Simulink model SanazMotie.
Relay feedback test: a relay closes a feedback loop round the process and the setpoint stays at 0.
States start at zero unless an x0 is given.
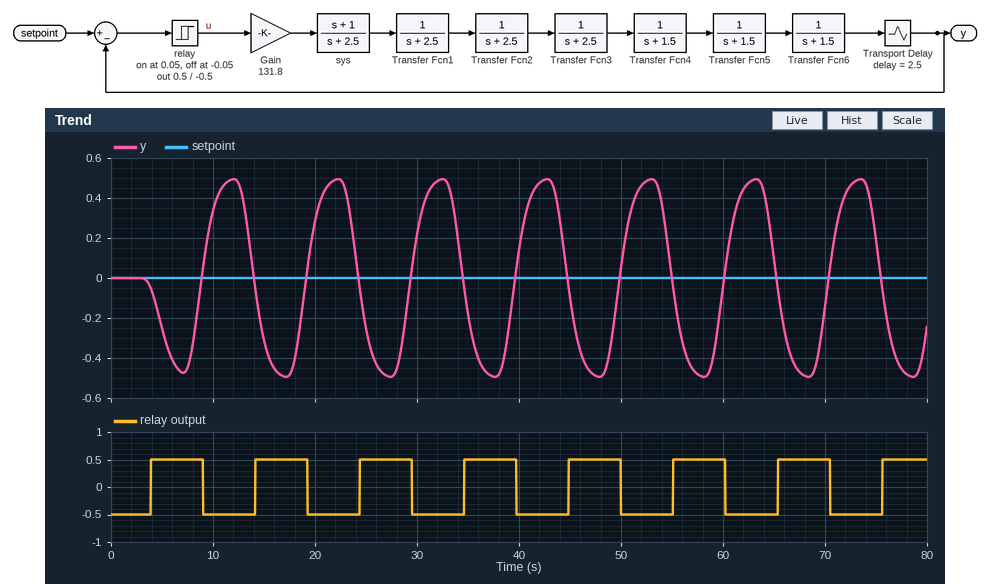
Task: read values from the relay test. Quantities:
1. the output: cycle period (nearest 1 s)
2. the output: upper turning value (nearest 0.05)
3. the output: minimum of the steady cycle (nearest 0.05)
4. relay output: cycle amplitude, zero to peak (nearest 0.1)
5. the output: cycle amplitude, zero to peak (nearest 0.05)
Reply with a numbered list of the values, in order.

1. 10 s
2. 0.50
3. -0.50
4. 0.5
5. 0.50
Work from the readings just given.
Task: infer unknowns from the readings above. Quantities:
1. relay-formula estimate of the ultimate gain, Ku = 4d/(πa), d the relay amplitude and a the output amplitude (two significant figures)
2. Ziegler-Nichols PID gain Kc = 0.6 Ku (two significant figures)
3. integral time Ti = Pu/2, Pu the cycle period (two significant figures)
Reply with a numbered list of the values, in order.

1. 1.3
2. 0.78
3. 5.0 s
